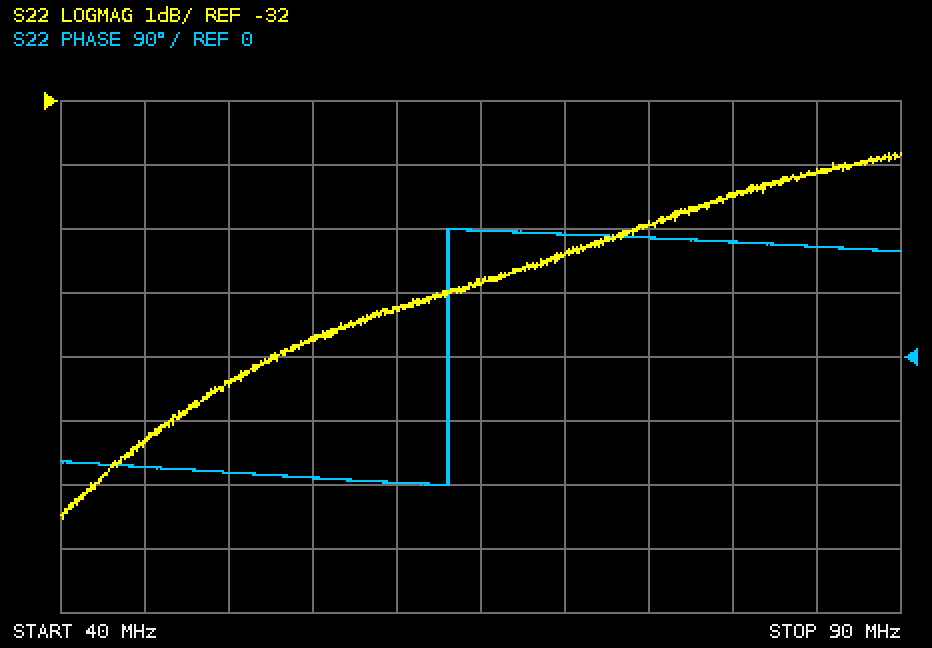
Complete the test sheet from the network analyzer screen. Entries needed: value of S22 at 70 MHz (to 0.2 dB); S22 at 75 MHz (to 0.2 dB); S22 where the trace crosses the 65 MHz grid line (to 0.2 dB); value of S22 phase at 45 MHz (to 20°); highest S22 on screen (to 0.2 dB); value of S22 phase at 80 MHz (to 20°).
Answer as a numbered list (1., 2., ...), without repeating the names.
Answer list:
1. -34.4 dB
2. -34.0 dB
3. -34.8 dB
4. -160°
5. -32.8 dB
6. 160°
